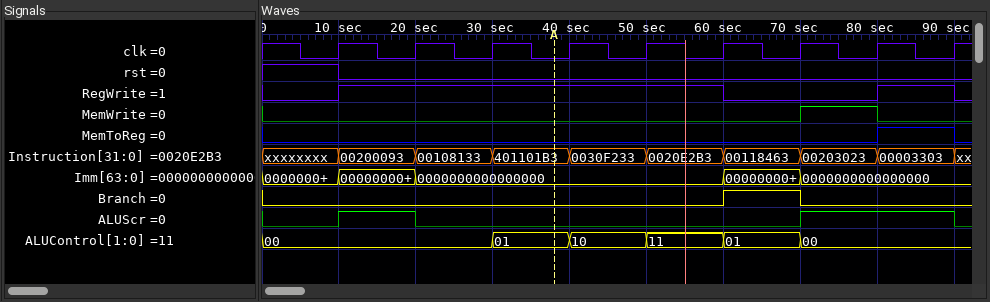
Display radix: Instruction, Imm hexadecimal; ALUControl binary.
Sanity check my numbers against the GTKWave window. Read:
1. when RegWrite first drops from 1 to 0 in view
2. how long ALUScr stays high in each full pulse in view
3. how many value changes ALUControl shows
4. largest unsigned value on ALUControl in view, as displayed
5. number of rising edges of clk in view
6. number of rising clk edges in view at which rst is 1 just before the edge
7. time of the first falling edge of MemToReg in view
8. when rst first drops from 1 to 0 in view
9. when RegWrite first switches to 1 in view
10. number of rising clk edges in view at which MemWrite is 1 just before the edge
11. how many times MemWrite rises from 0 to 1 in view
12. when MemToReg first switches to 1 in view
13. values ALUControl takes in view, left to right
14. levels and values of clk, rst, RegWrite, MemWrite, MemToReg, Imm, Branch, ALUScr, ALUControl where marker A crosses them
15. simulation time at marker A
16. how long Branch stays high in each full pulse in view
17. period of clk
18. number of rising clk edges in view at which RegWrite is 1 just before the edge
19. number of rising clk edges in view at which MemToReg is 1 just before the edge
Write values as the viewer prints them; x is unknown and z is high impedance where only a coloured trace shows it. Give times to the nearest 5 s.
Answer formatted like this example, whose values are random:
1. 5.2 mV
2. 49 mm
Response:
1. 60 s
2. 10 s, 20 s
3. 5
4. 11
5. 9
6. 1
7. 90 s
8. 10 s
9. 10 s
10. 1
11. 1
12. 80 s
13. 00, 01, 10, 11, 01, 00
14. clk=0, rst=0, RegWrite=1, MemWrite=0, MemToReg=0, Imm=0000000000000000, Branch=0, ALUScr=0, ALUControl=01
15. 40 s
16. 10 s
17. 10 s
18. 6
19. 1
